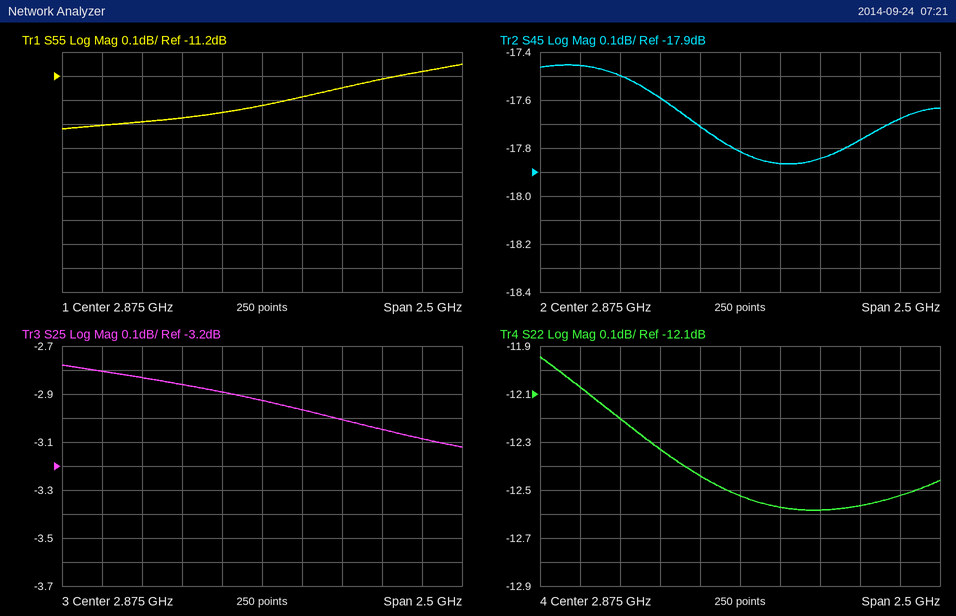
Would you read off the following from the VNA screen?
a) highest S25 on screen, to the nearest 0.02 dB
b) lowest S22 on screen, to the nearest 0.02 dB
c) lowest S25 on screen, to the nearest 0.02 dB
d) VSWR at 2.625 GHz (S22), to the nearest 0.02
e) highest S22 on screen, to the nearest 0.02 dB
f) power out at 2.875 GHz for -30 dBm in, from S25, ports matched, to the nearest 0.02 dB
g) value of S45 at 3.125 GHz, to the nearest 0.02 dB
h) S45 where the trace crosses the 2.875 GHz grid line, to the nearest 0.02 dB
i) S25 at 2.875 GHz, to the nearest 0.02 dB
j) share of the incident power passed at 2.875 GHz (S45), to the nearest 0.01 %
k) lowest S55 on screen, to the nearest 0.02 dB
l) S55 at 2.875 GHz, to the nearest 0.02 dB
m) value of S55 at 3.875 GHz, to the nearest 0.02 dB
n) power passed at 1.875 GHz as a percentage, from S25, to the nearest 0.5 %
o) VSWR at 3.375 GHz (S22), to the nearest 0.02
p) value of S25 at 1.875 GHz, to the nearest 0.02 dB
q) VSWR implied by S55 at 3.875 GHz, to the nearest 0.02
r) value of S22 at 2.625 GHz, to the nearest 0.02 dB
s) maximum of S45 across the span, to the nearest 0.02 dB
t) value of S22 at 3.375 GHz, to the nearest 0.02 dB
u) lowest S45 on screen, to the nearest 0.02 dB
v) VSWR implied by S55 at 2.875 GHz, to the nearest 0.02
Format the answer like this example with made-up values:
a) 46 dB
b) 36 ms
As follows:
a) -2.78 dB
b) -12.58 dB
c) -3.12 dB
d) 1.62
e) -11.94 dB
f) -32.92 dBm
g) -17.86 dB
h) -17.82 dB
i) -2.92 dB
j) 1.65 %
k) -11.42 dB
l) -11.32 dB
m) -11.18 dB
n) 52.5 %
o) 1.62
p) -2.80 dB
q) 1.76
r) -12.44 dB
s) -17.46 dB
t) -12.58 dB
u) -17.86 dB
v) 1.74
